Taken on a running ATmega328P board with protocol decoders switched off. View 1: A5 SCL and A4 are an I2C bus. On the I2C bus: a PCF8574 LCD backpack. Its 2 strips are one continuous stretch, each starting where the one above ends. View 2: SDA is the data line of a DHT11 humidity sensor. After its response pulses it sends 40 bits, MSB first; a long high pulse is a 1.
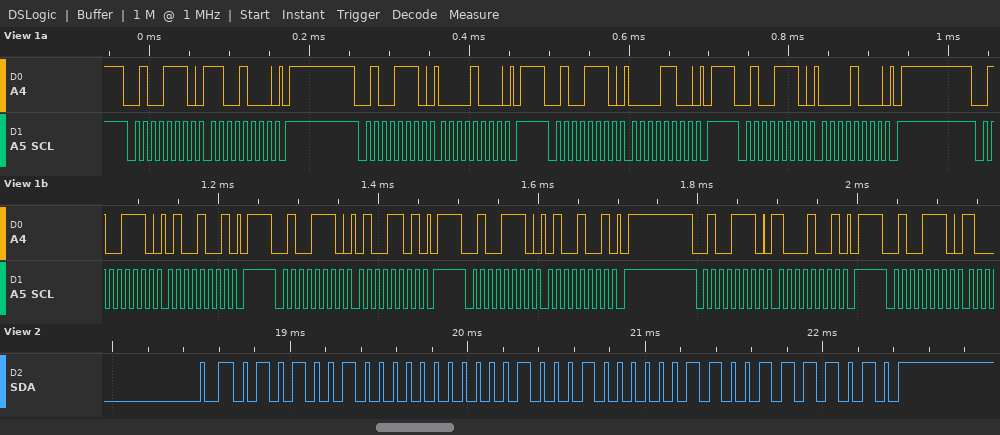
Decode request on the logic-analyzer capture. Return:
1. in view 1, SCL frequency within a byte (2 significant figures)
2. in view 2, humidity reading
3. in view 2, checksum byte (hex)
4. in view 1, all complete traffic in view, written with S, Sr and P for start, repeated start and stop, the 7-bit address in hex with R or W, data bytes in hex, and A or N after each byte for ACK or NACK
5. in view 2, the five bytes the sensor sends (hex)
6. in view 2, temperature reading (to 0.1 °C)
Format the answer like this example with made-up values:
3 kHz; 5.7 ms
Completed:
100 kHz; 82 %; 0x7A; S 27W A C8 A P S 27W A 08 A P S 27W A 0C A P S 27W A 08 A P S 27W A 49 A P S 27W A 4D A P S 27W A 49 A P S 27W A 89 A P S 27W A; 52 00 22 06 7A; 34.6 °C
